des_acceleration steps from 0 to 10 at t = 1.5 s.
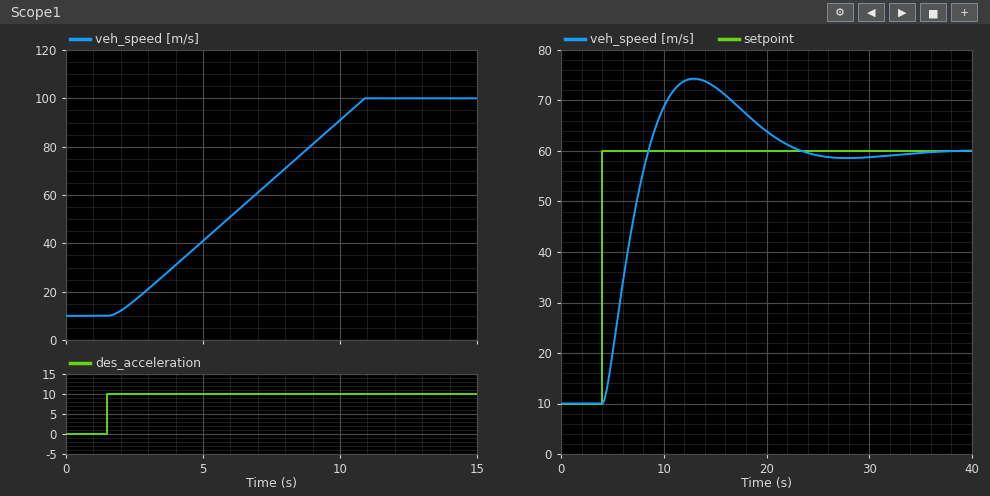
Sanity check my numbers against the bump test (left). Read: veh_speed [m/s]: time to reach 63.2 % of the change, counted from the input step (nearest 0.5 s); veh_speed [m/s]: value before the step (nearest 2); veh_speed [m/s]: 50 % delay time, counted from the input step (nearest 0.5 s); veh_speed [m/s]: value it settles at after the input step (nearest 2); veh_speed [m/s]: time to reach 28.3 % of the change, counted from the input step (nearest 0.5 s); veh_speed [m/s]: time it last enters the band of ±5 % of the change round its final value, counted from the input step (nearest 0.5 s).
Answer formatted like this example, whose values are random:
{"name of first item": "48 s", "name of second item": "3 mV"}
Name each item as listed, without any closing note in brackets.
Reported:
{"veh_speed [m/s]: time to reach 63.2 % of the change, counted from the input step": "6.0 s", "veh_speed [m/s]: value before the step": "10", "veh_speed [m/s]: 50 % delay time, counted from the input step": "5.0 s", "veh_speed [m/s]: value it settles at after the input step": "100", "veh_speed [m/s]: time to reach 28.3 % of the change, counted from the input step": "3.0 s", "veh_speed [m/s]: time it last enters the band of ±5 % of the change round its final value, counted from the input step": "9.0 s"}
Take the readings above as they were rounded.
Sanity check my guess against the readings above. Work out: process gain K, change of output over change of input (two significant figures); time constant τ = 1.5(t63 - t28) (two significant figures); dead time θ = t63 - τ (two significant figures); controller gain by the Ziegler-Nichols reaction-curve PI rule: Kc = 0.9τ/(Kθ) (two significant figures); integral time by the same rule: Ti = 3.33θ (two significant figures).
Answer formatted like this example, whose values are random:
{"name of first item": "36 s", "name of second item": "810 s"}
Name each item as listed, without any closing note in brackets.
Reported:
{"process gain K, change of output over change of input": "9.0", "time constant τ = 1.5(t63 - t28)": "4.5 s", "dead time θ = t63 - τ": "1.5 s", "controller gain by the Ziegler-Nichols reaction-curve PI rule: Kc = 0.9τ/(Kθ)": "0.30", "integral time by the same rule: Ti = 3.33θ": "5.0 s"}
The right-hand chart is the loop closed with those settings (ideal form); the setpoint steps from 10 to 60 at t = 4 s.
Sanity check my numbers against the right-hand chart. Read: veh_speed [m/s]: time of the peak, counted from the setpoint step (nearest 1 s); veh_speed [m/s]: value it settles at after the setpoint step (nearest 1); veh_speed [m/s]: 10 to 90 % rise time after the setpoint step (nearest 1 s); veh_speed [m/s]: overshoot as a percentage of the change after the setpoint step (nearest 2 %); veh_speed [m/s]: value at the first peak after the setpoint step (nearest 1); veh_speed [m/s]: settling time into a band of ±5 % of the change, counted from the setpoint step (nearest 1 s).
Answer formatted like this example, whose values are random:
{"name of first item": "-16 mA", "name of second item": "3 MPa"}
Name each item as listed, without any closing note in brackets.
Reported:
{"veh_speed [m/s]: time of the peak, counted from the setpoint step": "9 s", "veh_speed [m/s]: value it settles at after the setpoint step": "60", "veh_speed [m/s]: 10 to 90 % rise time after the setpoint step": "3 s", "veh_speed [m/s]: overshoot as a percentage of the change after the setpoint step": "28 %", "veh_speed [m/s]: value at the first peak after the setpoint step": "74", "veh_speed [m/s]: settling time into a band of ±5 % of the change, counted from the setpoint step": "17 s"}
